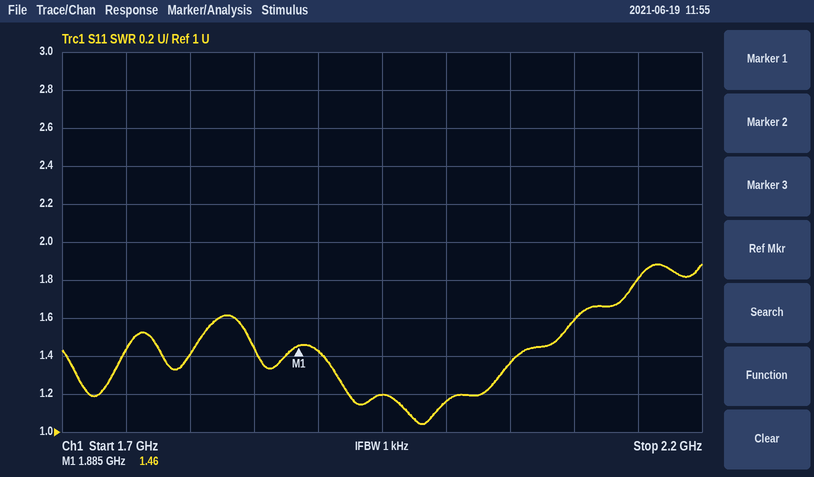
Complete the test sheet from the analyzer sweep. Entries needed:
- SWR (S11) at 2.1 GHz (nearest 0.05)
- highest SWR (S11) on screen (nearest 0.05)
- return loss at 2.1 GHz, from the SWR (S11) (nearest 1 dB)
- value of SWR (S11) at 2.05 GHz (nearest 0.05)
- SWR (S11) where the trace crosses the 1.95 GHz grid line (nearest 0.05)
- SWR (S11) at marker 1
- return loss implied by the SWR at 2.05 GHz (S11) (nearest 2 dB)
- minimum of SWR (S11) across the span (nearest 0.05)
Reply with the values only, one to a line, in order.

1.60
1.90
13 dB
1.35
1.20
1.46
16 dB
1.05
